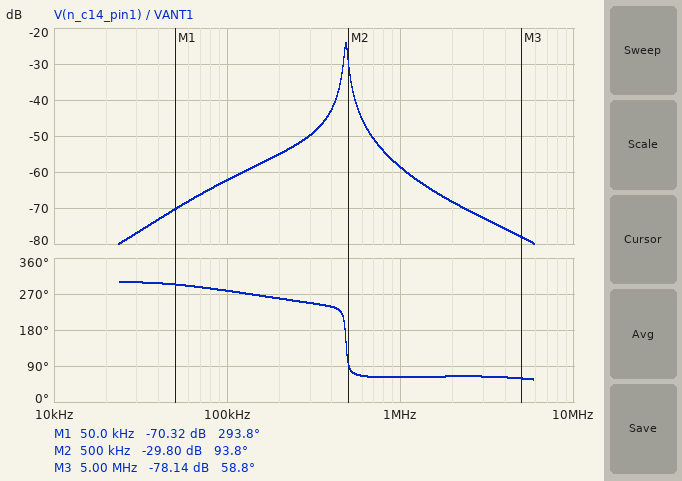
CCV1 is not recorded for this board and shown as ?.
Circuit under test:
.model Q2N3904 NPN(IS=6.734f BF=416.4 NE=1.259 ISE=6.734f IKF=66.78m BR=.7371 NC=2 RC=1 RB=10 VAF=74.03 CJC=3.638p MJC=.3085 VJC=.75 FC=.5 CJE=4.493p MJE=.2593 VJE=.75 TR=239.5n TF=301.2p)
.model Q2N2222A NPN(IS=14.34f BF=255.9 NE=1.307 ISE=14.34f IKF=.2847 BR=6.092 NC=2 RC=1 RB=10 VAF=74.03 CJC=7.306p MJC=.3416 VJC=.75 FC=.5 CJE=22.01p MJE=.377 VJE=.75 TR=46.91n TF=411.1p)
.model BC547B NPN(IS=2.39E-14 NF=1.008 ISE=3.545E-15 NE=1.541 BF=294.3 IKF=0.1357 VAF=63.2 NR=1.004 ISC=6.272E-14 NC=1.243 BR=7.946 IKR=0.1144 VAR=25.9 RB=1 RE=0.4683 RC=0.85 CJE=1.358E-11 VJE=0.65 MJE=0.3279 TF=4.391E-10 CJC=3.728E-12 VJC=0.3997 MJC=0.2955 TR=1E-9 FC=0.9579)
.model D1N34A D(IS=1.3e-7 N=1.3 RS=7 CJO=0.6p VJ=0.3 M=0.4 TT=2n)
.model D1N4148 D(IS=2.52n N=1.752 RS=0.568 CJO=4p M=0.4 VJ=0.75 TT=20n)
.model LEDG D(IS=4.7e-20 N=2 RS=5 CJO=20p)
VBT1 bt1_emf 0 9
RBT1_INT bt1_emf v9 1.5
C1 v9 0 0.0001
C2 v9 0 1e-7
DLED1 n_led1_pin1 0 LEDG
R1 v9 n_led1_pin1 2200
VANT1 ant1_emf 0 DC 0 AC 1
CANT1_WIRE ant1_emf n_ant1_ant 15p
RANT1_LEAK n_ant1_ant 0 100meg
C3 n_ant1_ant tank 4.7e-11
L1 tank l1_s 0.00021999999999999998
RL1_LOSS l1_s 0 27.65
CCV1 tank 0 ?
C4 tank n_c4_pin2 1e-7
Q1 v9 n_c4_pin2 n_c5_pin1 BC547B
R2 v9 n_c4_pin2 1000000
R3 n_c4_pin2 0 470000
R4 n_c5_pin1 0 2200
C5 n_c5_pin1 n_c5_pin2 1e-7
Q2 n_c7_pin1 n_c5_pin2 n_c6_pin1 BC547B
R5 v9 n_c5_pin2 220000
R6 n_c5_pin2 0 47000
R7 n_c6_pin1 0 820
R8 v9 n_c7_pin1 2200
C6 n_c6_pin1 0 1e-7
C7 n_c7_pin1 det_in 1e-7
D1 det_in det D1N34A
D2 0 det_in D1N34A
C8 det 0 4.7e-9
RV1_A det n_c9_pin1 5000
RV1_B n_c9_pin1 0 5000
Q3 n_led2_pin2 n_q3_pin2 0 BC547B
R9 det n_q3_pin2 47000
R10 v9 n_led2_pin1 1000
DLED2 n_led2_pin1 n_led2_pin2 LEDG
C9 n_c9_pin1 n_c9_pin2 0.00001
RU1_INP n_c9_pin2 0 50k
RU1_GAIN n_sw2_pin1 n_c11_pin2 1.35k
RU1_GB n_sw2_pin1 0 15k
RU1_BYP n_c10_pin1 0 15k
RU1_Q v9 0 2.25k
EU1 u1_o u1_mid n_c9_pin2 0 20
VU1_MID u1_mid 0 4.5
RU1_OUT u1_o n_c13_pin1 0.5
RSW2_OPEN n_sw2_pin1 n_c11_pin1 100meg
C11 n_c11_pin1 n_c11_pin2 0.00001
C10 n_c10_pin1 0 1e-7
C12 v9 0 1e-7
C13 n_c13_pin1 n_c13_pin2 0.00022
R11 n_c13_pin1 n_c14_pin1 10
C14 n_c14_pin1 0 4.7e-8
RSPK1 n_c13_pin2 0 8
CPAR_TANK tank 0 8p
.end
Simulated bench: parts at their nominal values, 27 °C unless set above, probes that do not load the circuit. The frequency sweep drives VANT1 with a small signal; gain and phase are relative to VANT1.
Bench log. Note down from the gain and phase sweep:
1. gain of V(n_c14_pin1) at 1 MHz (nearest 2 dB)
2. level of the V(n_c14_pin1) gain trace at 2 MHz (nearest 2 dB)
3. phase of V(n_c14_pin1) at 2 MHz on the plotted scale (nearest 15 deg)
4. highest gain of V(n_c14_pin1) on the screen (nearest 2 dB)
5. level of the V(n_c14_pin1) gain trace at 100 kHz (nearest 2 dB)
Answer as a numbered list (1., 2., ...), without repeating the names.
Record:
1. -58 dB
2. -68 dB
3. 60 deg
4. -24 dB
5. -62 dB
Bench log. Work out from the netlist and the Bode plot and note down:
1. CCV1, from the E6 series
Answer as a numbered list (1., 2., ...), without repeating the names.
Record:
1. 470 pF
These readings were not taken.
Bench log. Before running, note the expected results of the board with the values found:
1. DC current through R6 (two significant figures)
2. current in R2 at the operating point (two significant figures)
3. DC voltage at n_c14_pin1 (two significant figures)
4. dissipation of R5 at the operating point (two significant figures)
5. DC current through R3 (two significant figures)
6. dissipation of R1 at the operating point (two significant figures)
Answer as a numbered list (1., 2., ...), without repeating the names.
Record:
1. 31 µA
2. 6.8 µA
3. 4.5 V
4. 260 µW
5. 4.6 µA
6. 22 mW
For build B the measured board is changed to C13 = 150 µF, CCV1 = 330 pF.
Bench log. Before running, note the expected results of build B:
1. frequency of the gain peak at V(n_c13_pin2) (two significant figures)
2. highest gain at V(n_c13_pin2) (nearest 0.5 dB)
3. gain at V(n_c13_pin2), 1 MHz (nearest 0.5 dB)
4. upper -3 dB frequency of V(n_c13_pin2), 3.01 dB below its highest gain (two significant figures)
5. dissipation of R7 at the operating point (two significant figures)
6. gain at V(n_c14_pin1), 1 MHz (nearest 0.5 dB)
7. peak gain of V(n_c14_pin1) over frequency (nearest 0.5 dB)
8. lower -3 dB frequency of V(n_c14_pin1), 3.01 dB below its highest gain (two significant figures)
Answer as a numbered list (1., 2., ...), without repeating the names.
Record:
1. 570 kHz
2. -16.0 dB
3. -45.0 dB
4. 580 kHz
5. 820 µW
6. -54.5 dB
7. -22.0 dB
8. 560 kHz
